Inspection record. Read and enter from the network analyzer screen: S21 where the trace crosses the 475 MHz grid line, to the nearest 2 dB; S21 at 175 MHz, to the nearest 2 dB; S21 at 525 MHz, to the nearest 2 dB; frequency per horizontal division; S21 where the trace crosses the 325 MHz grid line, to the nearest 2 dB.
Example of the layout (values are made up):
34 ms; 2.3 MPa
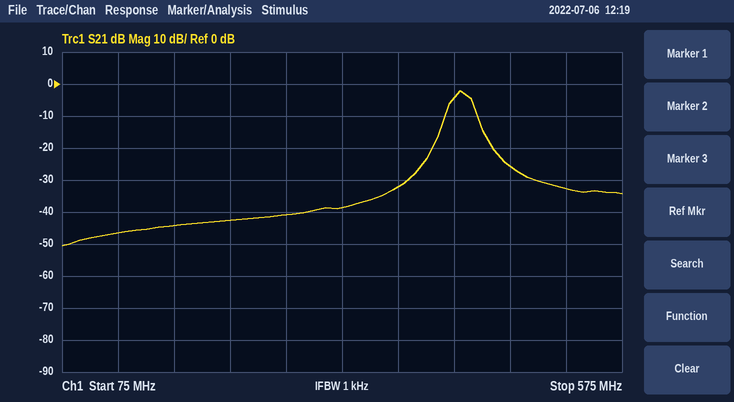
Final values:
-26 dB; -44 dB; -32 dB; 50 MHz; -38 dB
